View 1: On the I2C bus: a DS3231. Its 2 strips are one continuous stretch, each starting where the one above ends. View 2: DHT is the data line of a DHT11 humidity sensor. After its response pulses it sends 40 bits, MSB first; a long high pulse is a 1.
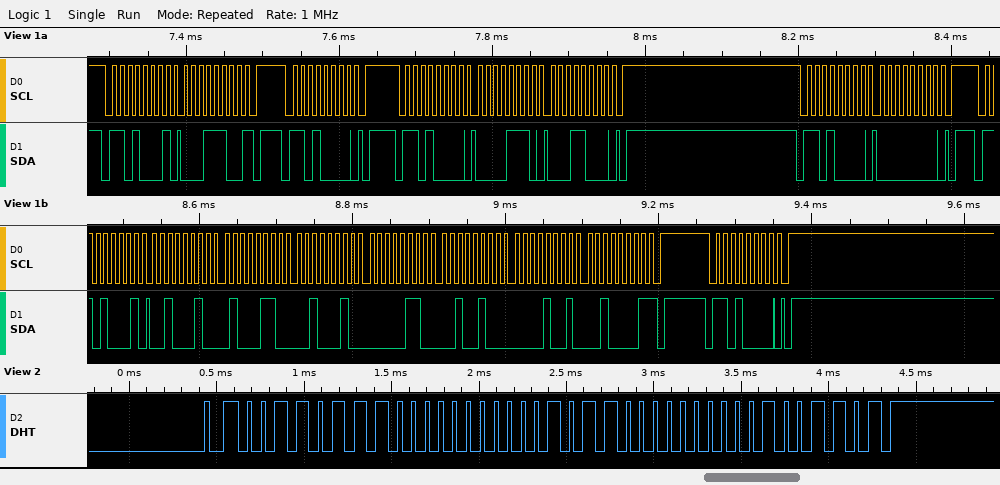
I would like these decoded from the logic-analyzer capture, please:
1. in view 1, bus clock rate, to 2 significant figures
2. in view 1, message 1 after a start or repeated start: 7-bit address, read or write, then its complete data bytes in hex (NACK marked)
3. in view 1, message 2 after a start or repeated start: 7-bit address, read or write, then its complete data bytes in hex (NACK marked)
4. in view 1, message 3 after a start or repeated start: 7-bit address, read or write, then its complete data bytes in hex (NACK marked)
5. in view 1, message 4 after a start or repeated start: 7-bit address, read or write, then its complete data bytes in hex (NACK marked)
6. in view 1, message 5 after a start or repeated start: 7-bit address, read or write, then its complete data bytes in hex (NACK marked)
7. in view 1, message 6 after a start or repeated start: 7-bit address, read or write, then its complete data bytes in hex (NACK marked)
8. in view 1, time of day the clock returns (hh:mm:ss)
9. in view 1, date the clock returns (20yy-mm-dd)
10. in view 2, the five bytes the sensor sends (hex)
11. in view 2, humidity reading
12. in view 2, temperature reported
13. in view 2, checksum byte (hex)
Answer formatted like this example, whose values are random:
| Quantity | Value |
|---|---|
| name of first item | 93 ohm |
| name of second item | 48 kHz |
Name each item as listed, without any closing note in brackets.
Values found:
| Quantity | Value |
|---|---|
| in view 1, bus clock rate, to 2 significant figures | 100 kHz |
| in view 1, message 1 after a start or repeated start: 7-bit address, read or write, then its complete data bytes in hex | 0x68 read: 1C NACK |
| in view 1, message 2 after a start or repeated start: 7-bit address, read or write, then its complete data bytes in hex | 0x68 write |
| in view 1, message 3 after a start or repeated start: 7-bit address, read or write, then its complete data bytes in hex | 0x68 write: 0E 18 |
| in view 1, message 4 after a start or repeated start: 7-bit address, read or write, then its complete data bytes in hex | 0x68 write: 00 |
| in view 1, message 5 after a start or repeated start: 7-bit address, read or write, then its complete data bytes in hex | 0x68 read: 22 46 22 06 24 09 21 NACK |
| in view 1, message 6 after a start or repeated start: 7-bit address, read or write, then its complete data bytes in hex | 0x68 write |
| in view 1, time of day the clock returns | 22:46:22 |
| in view 1, date the clock returns | 2021-09-24 |
| in view 2, the five bytes the sensor sends | 37 00 16 00 4D |
| in view 2, humidity reading | 55 % |
| in view 2, temperature reported | 22.0 °C |
| in view 2, checksum byte | 0x4D |
